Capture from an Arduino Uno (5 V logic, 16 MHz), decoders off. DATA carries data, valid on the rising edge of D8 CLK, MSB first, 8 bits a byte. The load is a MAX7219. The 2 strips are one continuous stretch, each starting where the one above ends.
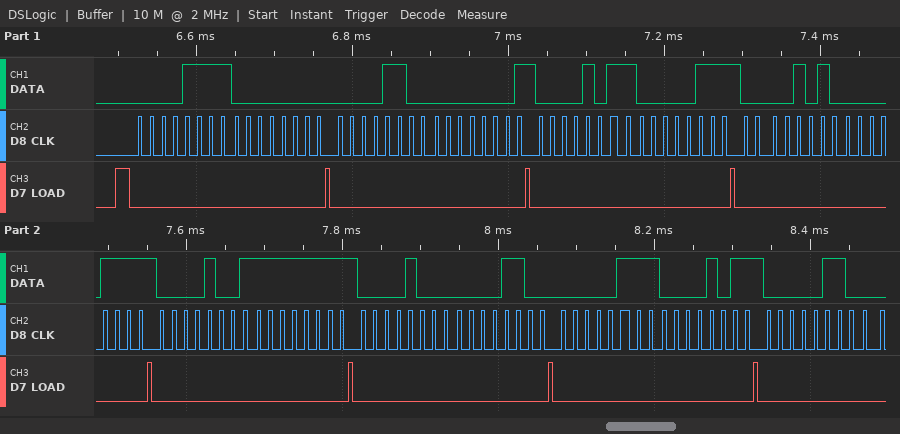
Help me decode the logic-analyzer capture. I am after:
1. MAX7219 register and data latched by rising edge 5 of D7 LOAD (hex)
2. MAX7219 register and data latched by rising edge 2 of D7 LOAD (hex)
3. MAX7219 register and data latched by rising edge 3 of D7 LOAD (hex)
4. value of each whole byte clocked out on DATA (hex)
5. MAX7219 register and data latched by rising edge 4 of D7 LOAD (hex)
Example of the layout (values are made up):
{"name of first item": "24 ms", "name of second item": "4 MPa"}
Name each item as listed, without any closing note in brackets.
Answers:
{"MAX7219 register and data latched by rising edge 5 of D7 LOAD": "register 0xA, data 0x0F", "MAX7219 register and data latched by rising edge 2 of D7 LOAD": "register 0xF, data 0x00", "MAX7219 register and data latched by rising edge 3 of D7 LOAD": "register 0xC, data 0x01", "value of each whole byte clocked out on DATA": "0F 00 0C 01 0B 07 0A 0F 09 FF 08 0C 07 0B 06", "MAX7219 register and data latched by rising edge 4 of D7 LOAD": "register 0xB, data 0x07"}
